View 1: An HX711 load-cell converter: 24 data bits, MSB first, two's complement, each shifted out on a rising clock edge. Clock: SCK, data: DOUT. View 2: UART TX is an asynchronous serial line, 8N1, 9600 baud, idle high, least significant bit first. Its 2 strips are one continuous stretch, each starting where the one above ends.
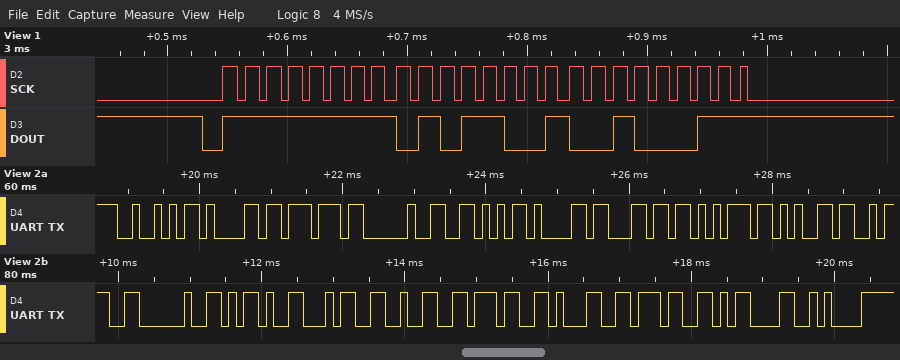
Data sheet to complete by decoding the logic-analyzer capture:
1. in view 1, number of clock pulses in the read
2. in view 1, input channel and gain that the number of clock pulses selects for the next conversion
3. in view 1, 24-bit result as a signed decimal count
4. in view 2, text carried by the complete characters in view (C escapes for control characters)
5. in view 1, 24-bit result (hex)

25
channel A, gain 128
-42717
"Raw Value: -42717\r\n"
0xFF5923
